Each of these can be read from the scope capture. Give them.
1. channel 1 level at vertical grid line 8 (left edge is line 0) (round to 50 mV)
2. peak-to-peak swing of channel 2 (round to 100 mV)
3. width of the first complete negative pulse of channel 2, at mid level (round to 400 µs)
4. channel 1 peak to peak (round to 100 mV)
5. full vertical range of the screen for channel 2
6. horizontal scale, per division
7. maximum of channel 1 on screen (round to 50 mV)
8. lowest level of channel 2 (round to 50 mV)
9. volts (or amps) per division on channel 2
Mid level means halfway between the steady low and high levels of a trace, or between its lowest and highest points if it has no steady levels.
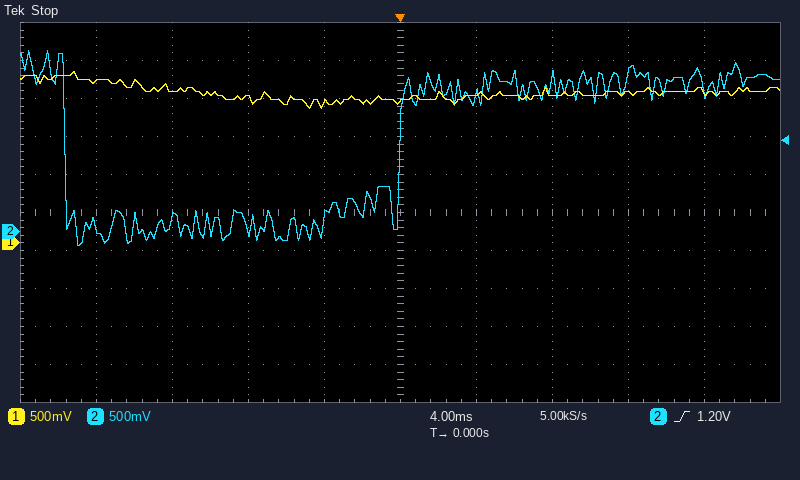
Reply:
1.95 V
2.60 V
17.6 ms
500 mV
5 V
4 ms
2.25 V
-200 mV
500 mV
